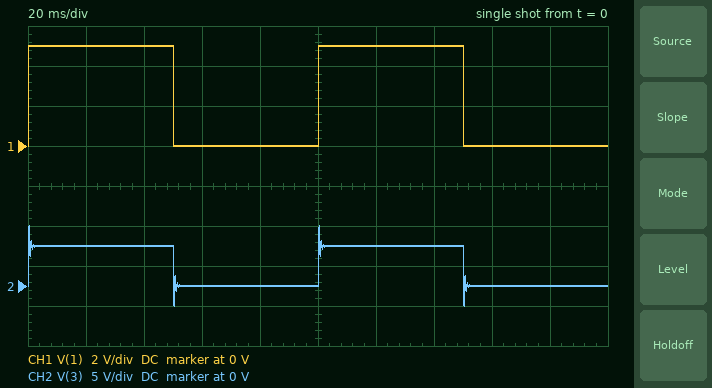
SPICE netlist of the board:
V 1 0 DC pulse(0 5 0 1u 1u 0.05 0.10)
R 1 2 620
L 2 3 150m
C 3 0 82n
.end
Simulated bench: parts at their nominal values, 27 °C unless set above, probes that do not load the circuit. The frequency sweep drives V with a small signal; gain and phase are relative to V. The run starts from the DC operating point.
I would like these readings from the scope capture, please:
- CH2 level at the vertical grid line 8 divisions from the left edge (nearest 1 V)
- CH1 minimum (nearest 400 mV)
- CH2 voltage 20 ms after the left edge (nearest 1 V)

0 V
0 V
5 V
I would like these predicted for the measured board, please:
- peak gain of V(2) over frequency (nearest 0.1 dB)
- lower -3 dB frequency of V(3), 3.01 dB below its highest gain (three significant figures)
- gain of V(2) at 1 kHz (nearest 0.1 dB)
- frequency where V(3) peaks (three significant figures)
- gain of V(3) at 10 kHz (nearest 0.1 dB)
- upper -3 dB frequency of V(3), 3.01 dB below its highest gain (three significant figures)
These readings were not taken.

0 dB
961 Hz
-1.4 dB
1.36 kHz
-33.6 dB
1.66 kHz
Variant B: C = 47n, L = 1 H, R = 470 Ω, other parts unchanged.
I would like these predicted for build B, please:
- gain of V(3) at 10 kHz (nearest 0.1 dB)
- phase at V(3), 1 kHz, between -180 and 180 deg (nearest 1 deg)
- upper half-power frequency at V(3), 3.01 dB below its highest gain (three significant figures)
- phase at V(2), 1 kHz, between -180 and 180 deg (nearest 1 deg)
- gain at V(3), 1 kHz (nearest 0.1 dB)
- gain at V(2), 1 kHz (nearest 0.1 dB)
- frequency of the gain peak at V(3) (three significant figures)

-45.3 dB
-171 deg
769 Hz
9 deg
1.2 dB
-0.1 dB
732 Hz
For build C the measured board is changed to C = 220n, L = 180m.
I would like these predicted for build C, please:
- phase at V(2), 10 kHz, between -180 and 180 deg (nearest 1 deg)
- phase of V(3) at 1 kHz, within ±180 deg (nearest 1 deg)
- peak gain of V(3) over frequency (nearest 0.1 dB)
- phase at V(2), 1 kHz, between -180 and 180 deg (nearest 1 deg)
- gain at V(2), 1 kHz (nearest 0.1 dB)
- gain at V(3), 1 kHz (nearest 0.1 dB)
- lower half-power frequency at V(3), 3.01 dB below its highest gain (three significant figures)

3 deg
-123 deg
3.8 dB
57 deg
-5.2 dB
-0.2 dB
278 Hz
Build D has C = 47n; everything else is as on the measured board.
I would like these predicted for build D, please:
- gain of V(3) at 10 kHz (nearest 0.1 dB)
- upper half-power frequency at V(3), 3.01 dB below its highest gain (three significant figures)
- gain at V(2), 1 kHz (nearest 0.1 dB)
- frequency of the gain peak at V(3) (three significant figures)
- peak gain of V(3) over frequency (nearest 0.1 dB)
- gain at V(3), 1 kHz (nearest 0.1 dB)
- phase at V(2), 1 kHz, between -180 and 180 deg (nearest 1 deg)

-28.6 dB
2.15 kHz
-0.3 dB
1.84 kHz
9.3 dB
2.6 dB
-14 deg
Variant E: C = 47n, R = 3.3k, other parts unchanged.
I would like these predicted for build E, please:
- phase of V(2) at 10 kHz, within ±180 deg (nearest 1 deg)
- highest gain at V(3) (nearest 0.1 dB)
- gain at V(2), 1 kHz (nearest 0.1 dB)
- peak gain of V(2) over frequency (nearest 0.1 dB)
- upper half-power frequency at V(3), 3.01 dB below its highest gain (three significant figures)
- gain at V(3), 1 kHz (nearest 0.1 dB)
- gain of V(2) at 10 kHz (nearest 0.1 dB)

20 deg
0 dB
-4.5 dB
0 dB
1.36 kHz
-1.7 dB
-0.5 dB
